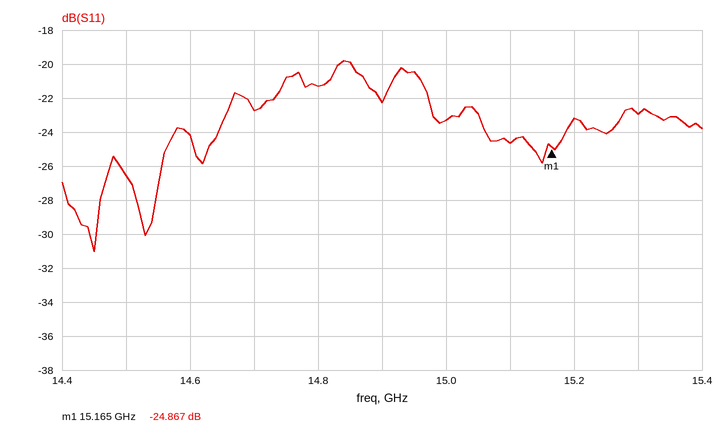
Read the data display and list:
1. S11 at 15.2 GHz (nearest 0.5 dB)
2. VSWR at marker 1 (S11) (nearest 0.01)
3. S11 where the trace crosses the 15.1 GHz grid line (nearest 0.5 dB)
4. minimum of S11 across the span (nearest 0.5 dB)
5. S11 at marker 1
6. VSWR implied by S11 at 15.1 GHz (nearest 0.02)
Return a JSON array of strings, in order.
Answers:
["-23.0 dB", "1.12", "-24.5 dB", "-31.0 dB", "-24.867 dB", "1.12"]
